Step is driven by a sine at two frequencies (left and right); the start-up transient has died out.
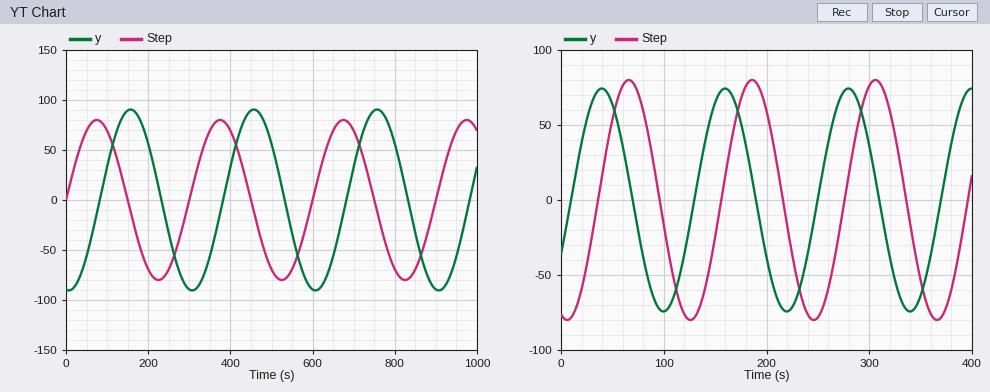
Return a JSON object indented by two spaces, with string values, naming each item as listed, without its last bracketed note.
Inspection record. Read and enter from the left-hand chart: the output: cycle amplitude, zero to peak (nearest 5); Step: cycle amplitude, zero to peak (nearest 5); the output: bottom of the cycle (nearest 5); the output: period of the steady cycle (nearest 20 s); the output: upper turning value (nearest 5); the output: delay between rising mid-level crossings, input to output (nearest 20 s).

{
  "the output: cycle amplitude, zero to peak": "90",
  "Step: cycle amplitude, zero to peak": "80",
  "the output: bottom of the cycle": "-90",
  "the output: period of the steady cycle": "300 s",
  "the output: upper turning value": "90",
  "the output: delay between rising mid-level crossings, input to output": "80 s"
}
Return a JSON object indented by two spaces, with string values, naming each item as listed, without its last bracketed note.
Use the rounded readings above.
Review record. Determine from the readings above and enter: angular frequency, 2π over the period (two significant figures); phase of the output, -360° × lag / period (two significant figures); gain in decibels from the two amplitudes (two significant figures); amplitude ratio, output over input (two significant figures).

{
  "angular frequency, 2π over the period": "0.021 rad/s",
  "phase of the output, -360° × lag / period": "-96°",
  "gain in decibels from the two amplitudes": "1.0 dB",
  "amplitude ratio, output over input": "1.1"
}
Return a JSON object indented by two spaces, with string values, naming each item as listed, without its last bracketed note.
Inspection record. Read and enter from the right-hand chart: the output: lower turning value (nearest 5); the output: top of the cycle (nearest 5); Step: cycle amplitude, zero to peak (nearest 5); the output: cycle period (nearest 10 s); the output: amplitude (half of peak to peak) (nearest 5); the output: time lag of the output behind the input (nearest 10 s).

{
  "the output: lower turning value": "-75",
  "the output: top of the cycle": "75",
  "Step: cycle amplitude, zero to peak": "80",
  "the output: cycle period": "120 s",
  "the output: amplitude (half of peak to peak)": "75",
  "the output: time lag of the output behind the input": "90 s"
}
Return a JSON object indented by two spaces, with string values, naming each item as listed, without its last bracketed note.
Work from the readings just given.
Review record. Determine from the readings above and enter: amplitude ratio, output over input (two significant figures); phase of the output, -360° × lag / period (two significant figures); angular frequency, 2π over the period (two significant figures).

{
  "amplitude ratio, output over input": "0.94",
  "phase of the output, -360° × lag / period": "-270°",
  "angular frequency, 2π over the period": "0.052 rad/s"
}
